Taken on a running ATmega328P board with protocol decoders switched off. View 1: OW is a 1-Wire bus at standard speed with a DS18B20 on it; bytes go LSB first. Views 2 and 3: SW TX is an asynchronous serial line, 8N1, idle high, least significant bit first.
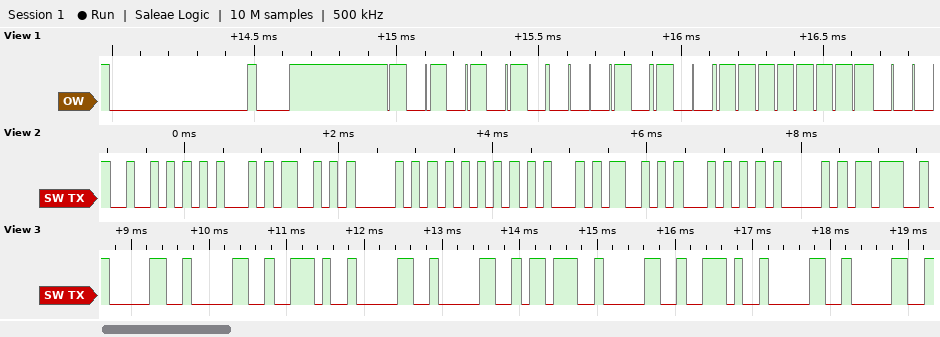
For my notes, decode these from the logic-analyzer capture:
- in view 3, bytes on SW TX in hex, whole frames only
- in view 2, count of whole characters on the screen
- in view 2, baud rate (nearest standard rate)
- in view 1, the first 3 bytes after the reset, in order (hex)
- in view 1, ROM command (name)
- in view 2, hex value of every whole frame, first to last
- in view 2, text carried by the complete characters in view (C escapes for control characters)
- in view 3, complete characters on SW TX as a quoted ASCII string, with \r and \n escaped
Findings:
30 30 2E 30 30 3B 30 2E 30 30
10
9600 baud
55 28 FF
Match ROM
0x52 0x45 0x53 0x50 0x55 0x45 0x53 0x54 0x41 0x3B
"RESPUESTA;"
"00.00;0.00"
